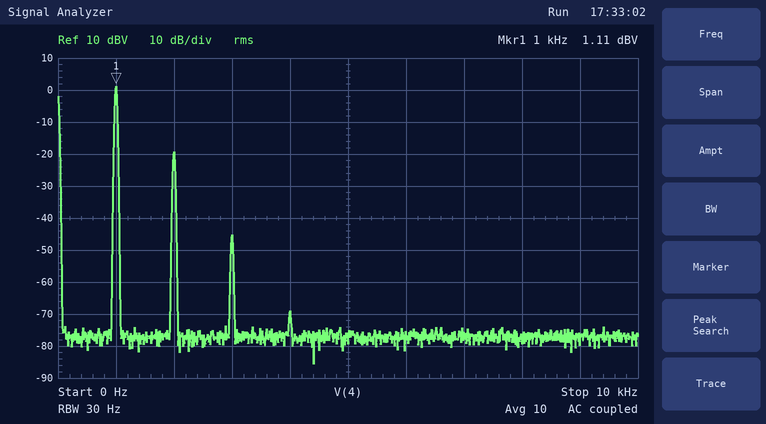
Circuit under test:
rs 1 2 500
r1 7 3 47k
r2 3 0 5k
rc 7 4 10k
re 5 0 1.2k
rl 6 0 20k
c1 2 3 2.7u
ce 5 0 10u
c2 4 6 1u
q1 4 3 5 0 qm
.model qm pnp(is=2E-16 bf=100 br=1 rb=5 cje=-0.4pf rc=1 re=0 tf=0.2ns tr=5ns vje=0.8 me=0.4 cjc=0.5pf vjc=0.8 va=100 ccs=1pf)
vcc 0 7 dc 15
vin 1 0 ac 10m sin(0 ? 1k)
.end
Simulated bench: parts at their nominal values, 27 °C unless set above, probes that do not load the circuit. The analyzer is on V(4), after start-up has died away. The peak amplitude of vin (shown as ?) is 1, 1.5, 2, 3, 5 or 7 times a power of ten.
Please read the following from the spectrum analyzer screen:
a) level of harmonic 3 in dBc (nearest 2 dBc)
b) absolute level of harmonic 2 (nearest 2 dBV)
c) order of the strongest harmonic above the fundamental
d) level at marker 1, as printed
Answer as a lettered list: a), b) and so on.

a) -46 dBc
b) -20 dBV
c) 2
d) 1.11 dBV
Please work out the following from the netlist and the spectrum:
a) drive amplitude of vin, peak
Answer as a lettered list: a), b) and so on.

a) 15 mV
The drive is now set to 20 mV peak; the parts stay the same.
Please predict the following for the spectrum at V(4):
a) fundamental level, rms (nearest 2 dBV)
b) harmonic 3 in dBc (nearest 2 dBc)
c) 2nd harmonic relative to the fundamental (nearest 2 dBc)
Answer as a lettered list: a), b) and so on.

a) 4 dBV
b) -42 dBc
c) -18 dBc
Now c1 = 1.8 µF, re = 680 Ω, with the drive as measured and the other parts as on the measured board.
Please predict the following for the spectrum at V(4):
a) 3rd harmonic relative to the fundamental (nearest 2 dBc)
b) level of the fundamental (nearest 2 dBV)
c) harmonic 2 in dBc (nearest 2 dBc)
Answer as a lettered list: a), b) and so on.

a) -52 dBc
b) 4 dBV
c) -22 dBc
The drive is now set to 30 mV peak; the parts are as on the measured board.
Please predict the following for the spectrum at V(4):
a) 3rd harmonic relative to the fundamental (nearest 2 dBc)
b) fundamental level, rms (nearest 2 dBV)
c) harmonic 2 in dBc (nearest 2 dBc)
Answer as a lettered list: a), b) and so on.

a) -34 dBc
b) 6 dBV
c) -14 dBc
